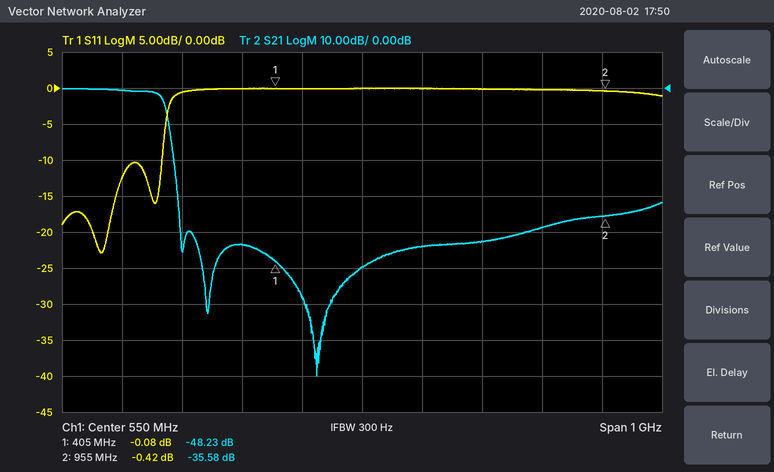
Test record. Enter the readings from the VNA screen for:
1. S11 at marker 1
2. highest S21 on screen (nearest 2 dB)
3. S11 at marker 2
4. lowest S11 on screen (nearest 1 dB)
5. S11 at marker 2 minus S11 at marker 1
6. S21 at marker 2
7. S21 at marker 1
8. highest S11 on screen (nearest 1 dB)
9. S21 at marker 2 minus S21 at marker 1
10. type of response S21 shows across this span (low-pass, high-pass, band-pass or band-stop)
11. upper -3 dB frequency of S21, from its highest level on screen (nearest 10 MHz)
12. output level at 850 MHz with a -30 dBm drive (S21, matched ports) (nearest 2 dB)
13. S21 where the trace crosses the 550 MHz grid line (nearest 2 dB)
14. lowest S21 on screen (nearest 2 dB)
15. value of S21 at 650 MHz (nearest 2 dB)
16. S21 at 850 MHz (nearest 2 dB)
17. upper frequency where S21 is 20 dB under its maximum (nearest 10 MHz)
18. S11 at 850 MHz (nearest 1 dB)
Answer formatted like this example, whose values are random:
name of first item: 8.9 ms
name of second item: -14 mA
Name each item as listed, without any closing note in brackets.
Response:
S11 at marker 1: -0.08 dB
highest S21 on screen: 0 dB
S11 at marker 2: -0.42 dB
lowest S11 on screen: -23 dB
S11 at marker 2 minus S11 at marker 1: -0.34 dB
S21 at marker 2: -35.58 dB
S21 at marker 1: -48.23 dB
highest S11 on screen: 0 dB
S21 at marker 2 minus S21 at marker 1: 12.65 dB
type of response S21 shows across this span: low-pass
upper -3 dB frequency of S21, from its highest level on screen: 220 MHz
output level at 850 MHz with a -30 dBm drive (S21, matched ports): -68 dBm
S21 where the trace crosses the 550 MHz grid line: -50 dB
lowest S21 on screen: -80 dB
value of S21 at 650 MHz: -44 dB
S21 at 850 MHz: -38 dB
upper frequency where S21 is 20 dB under its maximum: 240 MHz
S11 at 850 MHz: 0 dB
